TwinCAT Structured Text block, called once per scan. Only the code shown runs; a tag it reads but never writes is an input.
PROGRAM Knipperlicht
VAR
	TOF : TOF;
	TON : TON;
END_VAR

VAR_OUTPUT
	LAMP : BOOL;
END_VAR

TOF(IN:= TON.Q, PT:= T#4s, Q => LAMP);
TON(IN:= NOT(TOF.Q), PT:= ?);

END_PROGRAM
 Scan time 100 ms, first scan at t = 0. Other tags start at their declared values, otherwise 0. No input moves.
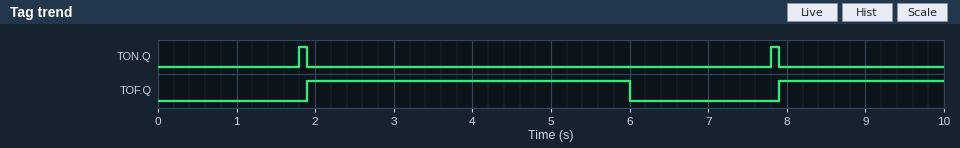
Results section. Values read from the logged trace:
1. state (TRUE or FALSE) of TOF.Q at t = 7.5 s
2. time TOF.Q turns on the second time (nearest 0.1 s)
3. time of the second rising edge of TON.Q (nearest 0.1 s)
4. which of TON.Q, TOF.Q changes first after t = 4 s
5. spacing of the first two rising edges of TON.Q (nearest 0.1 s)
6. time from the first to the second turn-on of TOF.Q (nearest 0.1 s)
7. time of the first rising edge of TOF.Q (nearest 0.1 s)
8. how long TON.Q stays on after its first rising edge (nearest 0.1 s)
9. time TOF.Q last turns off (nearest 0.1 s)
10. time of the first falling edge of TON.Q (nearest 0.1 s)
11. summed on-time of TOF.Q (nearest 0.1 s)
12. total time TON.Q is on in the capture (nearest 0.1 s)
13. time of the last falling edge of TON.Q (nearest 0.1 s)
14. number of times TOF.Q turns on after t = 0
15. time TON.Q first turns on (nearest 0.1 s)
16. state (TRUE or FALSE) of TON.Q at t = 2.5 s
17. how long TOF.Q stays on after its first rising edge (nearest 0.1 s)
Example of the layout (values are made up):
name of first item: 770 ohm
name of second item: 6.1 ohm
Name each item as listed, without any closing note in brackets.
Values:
state (TRUE or FALSE) of TOF.Q at t = 7.5 s: FALSE
time TOF.Q turns on the second time: 7.9 s
time of the second rising edge of TON.Q: 7.8 s
which of TON.Q, TOF.Q changes first after t = 4 s: TOF.Q
spacing of the first two rising edges of TON.Q: 6.0 s
time from the first to the second turn-on of TOF.Q: 6.0 s
time of the first rising edge of TOF.Q: 1.9 s
how long TON.Q stays on after its first rising edge: 0.1 s
time TOF.Q last turns off: 6.0 s
time of the first falling edge of TON.Q: 1.9 s
summed on-time of TOF.Q: 6.2 s
total time TON.Q is on in the capture: 0.2 s
time of the last falling edge of TON.Q: 7.9 s
number of times TOF.Q turns on after t = 0: 2
time TON.Q first turns on: 1.8 s
state (TRUE or FALSE) of TON.Q at t = 2.5 s: FALSE
how long TOF.Q stays on after its first rising edge: 4.1 s
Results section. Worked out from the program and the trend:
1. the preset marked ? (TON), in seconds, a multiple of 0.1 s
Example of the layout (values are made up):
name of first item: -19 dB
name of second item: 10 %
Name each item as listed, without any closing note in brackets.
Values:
the preset marked ? (TON), in seconds, a multiple of 0.1 s: 1.8 s
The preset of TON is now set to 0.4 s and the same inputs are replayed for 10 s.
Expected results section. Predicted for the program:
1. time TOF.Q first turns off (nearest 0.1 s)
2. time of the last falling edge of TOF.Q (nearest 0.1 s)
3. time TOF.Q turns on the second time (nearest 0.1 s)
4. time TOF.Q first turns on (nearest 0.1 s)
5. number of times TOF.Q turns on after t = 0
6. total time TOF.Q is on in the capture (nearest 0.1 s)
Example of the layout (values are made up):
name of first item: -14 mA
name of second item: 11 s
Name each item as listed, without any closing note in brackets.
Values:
time TOF.Q first turns off: 4.6 s
time of the last falling edge of TOF.Q: 9.2 s
time TOF.Q turns on the second time: 5.1 s
time TOF.Q first turns on: 0.5 s
number of times TOF.Q turns on after t = 0: 3
total time TOF.Q is on in the capture: 8.5 s
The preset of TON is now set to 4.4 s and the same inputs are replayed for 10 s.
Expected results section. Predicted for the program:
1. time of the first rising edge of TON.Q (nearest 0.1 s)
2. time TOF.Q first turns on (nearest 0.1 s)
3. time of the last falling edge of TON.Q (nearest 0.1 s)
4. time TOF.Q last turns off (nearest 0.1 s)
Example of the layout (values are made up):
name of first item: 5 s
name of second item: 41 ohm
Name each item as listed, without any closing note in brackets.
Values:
time of the first rising edge of TON.Q: 4.4 s
time TOF.Q first turns on: 4.5 s
time of the last falling edge of TON.Q: 4.5 s
time TOF.Q last turns off: 8.6 s
